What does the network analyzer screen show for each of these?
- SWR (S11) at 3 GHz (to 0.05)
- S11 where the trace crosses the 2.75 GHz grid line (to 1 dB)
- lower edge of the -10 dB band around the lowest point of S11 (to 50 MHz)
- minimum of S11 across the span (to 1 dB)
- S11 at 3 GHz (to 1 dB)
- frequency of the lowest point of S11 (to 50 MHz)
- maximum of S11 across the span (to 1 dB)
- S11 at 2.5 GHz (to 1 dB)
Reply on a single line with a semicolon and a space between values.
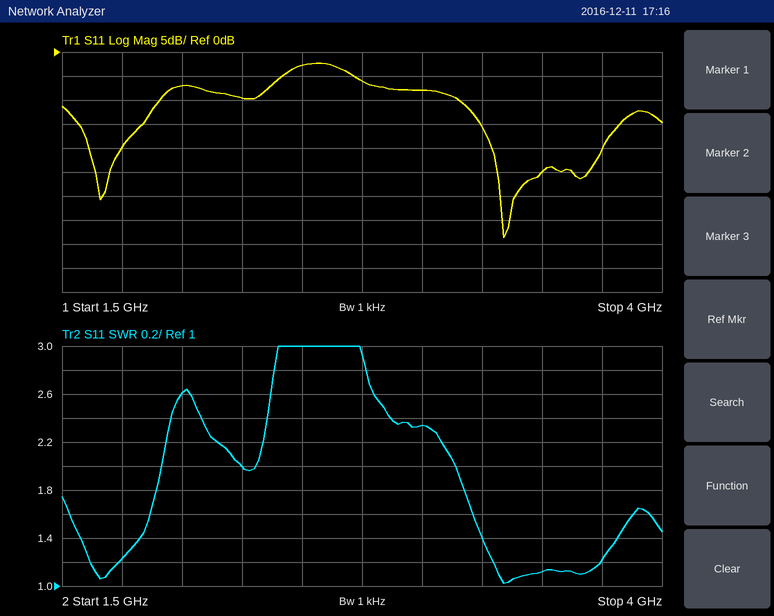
2.35; -6 dB; 3.15 GHz; -39 dB; -8 dB; 3.35 GHz; -2 dB; -3 dB
